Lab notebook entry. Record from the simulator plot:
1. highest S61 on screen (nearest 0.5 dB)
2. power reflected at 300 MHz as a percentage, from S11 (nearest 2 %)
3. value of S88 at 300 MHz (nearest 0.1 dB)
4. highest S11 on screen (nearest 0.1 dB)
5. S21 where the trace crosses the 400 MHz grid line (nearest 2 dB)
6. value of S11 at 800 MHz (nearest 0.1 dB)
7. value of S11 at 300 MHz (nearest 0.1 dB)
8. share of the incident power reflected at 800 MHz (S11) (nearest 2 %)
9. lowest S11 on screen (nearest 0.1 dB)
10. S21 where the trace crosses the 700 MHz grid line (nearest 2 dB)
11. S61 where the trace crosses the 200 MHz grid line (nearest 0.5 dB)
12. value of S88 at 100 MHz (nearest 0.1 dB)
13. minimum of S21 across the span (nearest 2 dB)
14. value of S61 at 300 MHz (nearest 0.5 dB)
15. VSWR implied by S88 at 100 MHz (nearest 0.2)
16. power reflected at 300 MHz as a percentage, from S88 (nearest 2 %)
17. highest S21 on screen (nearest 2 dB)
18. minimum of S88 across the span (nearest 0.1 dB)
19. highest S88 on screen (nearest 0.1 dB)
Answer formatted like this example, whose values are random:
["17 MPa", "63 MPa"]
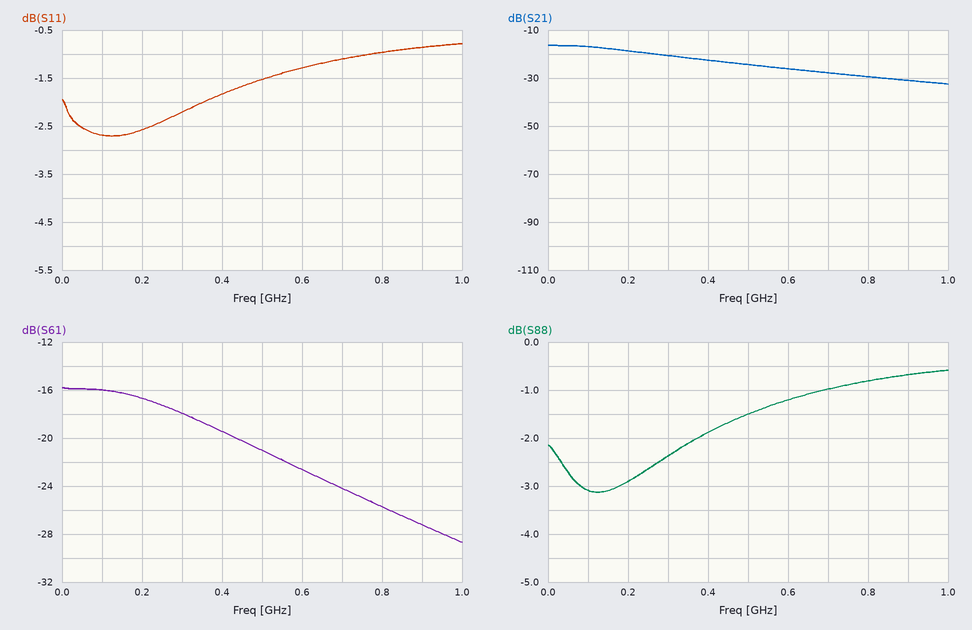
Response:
["-16.0 dB", "60 %", "-2.4 dB", "-0.8 dB", "-22 dB", "-1.0 dB", "-2.2 dB", "80 %", "-2.7 dB", "-28 dB", "-16.5 dB", "-3.1 dB", "-32 dB", "-18.0 dB", "5.6", "58 %", "-16 dB", "-3.1 dB", "-0.6 dB"]
